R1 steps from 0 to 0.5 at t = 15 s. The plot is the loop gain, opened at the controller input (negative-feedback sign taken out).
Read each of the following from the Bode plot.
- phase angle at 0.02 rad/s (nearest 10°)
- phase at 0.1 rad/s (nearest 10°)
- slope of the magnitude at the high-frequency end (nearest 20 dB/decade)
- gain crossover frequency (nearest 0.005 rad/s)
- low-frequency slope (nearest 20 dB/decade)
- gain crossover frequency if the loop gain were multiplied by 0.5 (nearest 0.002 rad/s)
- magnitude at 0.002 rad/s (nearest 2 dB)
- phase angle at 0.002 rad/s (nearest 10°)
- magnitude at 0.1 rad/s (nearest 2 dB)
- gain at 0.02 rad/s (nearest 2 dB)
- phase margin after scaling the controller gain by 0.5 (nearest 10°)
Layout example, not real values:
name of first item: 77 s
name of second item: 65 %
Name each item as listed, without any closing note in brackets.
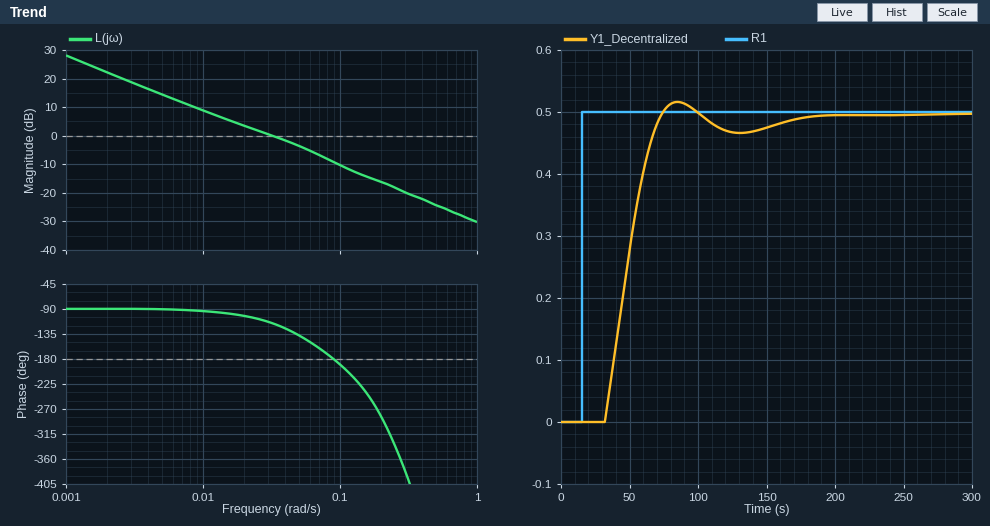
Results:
phase angle at 0.02 rad/s: -100°
phase at 0.1 rad/s: -190°
slope of the magnitude at the high-frequency end: -20 dB/decade
gain crossover frequency: 0.030 rad/s
low-frequency slope: -20 dB/decade
gain crossover frequency if the loop gain were multiplied by 0.5: 0.014 rad/s
magnitude at 0.002 rad/s: 22 dB
phase angle at 0.002 rad/s: -90°
magnitude at 0.1 rad/s: -10 dB
gain at 0.02 rad/s: 4 dB
phase margin after scaling the controller gain by 0.5: 80°
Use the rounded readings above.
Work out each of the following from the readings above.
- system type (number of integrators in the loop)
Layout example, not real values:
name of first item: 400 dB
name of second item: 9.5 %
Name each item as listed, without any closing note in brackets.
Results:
system type: 1
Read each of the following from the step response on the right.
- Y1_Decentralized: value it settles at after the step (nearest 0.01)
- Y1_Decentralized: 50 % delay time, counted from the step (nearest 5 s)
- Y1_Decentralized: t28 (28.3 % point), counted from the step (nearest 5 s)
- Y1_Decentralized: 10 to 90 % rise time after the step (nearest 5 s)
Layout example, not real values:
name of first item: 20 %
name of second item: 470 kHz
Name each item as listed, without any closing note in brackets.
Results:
Y1_Decentralized: value it settles at after the step: 0.50
Y1_Decentralized: 50 % delay time, counted from the step: 35 s
Y1_Decentralized: t28 (28.3 % point), counted from the step: 25 s
Y1_Decentralized: 10 to 90 % rise time after the step: 30 s
